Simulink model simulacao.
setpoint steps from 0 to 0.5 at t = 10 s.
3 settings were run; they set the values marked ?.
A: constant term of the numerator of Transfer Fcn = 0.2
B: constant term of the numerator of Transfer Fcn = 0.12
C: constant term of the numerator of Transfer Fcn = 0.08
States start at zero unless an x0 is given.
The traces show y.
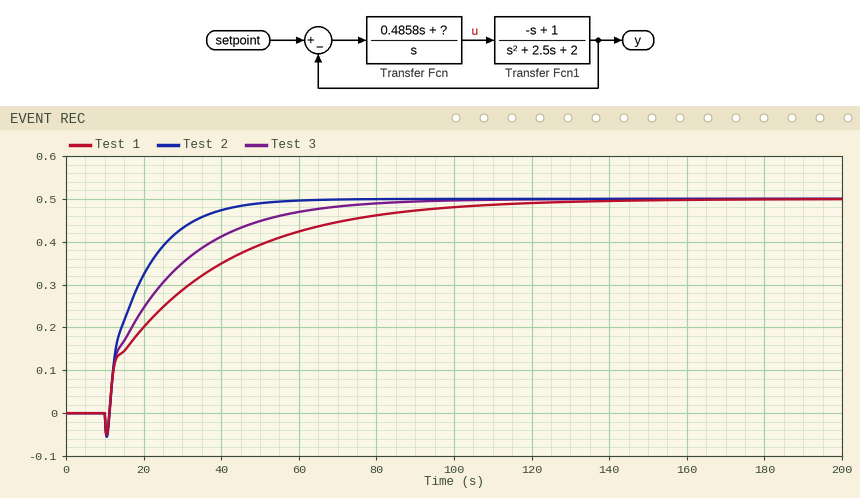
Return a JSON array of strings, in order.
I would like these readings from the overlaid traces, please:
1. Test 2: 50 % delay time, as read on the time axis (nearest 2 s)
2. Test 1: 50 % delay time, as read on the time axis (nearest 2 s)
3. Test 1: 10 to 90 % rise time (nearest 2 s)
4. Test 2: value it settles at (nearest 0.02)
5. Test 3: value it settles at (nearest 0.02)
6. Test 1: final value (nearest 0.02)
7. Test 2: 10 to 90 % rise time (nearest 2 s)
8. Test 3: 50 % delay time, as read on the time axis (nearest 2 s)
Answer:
["16 s", "26 s", "60 s", "0.50", "0.50", "0.50", "22 s", "20 s"]
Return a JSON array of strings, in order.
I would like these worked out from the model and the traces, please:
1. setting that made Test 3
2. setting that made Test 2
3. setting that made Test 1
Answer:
["B", "A", "C"]
